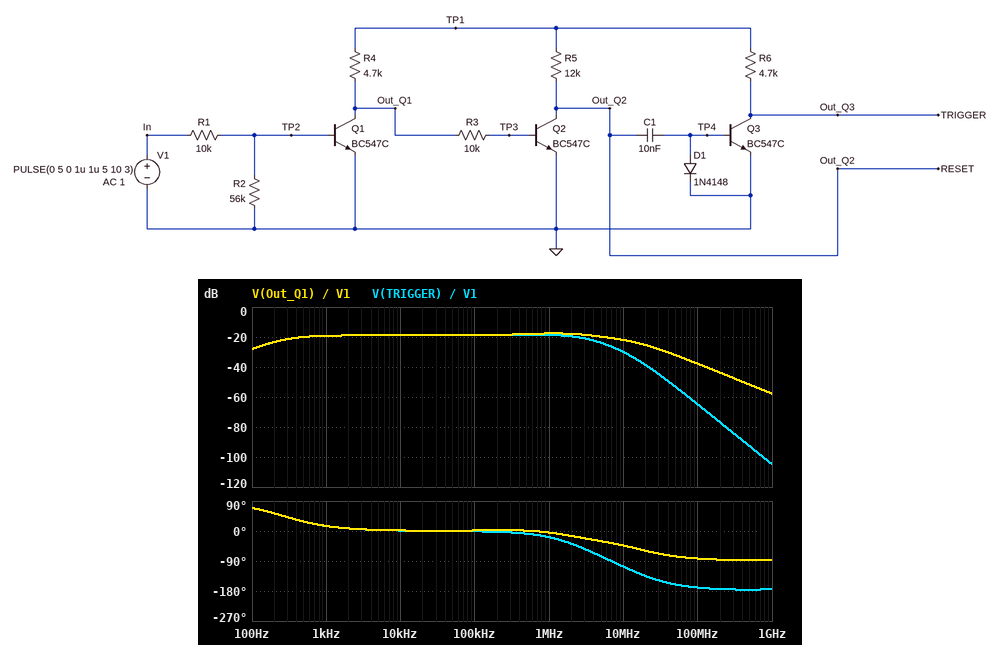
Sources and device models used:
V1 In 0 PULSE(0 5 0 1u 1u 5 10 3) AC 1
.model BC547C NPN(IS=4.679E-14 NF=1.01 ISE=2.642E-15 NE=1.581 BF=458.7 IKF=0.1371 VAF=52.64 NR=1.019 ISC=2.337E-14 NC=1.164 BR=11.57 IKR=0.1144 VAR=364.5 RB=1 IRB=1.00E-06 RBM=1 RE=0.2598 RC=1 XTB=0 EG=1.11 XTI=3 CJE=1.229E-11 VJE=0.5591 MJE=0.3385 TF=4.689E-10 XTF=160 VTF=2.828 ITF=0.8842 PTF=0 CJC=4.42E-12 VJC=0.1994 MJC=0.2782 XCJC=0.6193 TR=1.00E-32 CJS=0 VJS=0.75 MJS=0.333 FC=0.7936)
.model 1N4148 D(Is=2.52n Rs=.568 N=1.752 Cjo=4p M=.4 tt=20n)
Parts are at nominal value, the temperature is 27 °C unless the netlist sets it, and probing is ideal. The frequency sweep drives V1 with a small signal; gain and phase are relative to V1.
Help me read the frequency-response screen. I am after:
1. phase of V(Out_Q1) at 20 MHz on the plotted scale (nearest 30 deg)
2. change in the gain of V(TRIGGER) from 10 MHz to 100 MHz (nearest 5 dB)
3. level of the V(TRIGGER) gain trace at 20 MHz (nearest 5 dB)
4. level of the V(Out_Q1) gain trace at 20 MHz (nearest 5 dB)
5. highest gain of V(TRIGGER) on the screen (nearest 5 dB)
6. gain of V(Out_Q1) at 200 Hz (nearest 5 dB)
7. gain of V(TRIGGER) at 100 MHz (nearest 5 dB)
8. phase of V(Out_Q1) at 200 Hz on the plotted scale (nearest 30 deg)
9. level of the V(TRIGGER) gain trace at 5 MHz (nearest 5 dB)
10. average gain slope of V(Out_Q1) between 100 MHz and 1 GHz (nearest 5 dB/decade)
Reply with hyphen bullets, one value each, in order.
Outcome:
- -60 deg
- -35 dB
- -40 dB
- -25 dB
- -20 dB
- -25 dB
- -65 dB
- 60 deg
- -25 dB
- -20 dB/decade
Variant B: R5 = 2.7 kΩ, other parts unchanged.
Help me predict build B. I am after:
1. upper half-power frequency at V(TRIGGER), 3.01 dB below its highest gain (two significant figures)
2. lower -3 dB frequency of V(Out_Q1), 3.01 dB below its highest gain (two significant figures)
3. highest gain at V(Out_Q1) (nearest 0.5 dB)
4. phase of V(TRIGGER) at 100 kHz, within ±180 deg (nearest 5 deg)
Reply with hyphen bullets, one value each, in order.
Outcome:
- 1.5 MHz
- 270 Hz
- -19.0 dB
- -5 deg
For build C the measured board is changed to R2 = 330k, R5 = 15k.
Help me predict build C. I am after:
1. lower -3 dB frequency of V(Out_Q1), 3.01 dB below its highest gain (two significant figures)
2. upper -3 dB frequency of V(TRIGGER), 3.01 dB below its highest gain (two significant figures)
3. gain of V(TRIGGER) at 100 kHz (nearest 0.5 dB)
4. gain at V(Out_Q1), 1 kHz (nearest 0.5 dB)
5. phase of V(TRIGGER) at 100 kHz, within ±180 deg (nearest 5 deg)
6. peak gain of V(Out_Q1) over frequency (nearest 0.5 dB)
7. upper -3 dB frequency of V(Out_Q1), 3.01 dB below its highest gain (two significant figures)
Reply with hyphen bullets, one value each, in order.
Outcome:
- 360 Hz
- 3.0 MHz
- -17.5 dB
- -18.0 dB
- 0 deg
- -16.5 dB
- 5.1 MHz
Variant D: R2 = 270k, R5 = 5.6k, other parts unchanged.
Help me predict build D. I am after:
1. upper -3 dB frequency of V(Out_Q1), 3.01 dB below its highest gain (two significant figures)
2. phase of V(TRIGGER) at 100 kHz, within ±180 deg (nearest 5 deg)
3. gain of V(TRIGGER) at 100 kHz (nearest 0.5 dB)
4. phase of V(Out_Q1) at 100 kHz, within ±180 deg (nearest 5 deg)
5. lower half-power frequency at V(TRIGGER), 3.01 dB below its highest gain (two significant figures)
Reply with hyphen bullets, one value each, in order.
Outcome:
- 6.3 MHz
- -5 deg
- -18.0 dB
- 0 deg
- 270 Hz
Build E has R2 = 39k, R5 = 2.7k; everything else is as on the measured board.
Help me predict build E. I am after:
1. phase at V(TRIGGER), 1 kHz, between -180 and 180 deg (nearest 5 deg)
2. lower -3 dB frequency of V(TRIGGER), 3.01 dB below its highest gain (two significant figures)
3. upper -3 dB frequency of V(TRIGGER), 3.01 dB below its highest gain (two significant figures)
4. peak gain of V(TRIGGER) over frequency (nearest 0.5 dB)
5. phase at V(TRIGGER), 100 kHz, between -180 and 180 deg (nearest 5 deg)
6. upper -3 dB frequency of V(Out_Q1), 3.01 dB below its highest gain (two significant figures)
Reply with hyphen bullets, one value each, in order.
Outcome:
- 15 deg
- 270 Hz
- 1.6 MHz
- -19.5 dB
- -5 deg
- 9.5 MHz
